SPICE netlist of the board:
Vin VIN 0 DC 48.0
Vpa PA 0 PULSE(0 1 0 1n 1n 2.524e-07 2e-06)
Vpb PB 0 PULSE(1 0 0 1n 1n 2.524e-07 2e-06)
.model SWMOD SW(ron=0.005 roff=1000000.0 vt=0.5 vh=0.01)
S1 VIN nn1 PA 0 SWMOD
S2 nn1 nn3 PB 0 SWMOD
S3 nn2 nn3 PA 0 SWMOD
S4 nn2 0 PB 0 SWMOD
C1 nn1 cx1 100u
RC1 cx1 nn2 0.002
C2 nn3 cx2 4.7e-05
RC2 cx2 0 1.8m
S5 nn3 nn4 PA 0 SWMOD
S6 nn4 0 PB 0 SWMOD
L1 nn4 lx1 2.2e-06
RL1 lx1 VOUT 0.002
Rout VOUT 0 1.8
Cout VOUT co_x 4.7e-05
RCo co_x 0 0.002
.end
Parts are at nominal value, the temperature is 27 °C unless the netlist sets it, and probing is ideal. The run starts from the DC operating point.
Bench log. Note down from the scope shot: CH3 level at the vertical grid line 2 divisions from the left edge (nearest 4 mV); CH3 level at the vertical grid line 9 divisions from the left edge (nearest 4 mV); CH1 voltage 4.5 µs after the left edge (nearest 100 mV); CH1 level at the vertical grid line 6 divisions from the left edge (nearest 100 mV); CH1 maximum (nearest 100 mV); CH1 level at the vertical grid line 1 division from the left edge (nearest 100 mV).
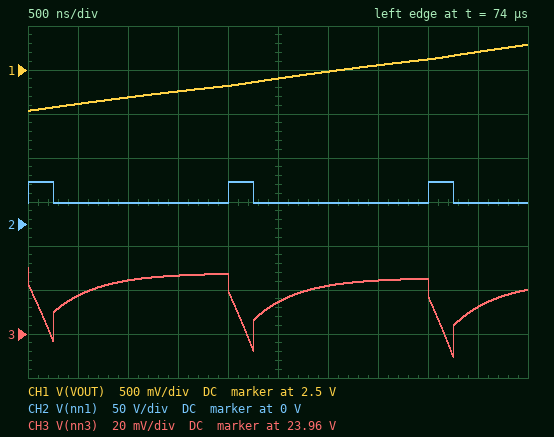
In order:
23.984 V
23.972 V
2.7 V
2.5 V
2.8 V
2.1 V
